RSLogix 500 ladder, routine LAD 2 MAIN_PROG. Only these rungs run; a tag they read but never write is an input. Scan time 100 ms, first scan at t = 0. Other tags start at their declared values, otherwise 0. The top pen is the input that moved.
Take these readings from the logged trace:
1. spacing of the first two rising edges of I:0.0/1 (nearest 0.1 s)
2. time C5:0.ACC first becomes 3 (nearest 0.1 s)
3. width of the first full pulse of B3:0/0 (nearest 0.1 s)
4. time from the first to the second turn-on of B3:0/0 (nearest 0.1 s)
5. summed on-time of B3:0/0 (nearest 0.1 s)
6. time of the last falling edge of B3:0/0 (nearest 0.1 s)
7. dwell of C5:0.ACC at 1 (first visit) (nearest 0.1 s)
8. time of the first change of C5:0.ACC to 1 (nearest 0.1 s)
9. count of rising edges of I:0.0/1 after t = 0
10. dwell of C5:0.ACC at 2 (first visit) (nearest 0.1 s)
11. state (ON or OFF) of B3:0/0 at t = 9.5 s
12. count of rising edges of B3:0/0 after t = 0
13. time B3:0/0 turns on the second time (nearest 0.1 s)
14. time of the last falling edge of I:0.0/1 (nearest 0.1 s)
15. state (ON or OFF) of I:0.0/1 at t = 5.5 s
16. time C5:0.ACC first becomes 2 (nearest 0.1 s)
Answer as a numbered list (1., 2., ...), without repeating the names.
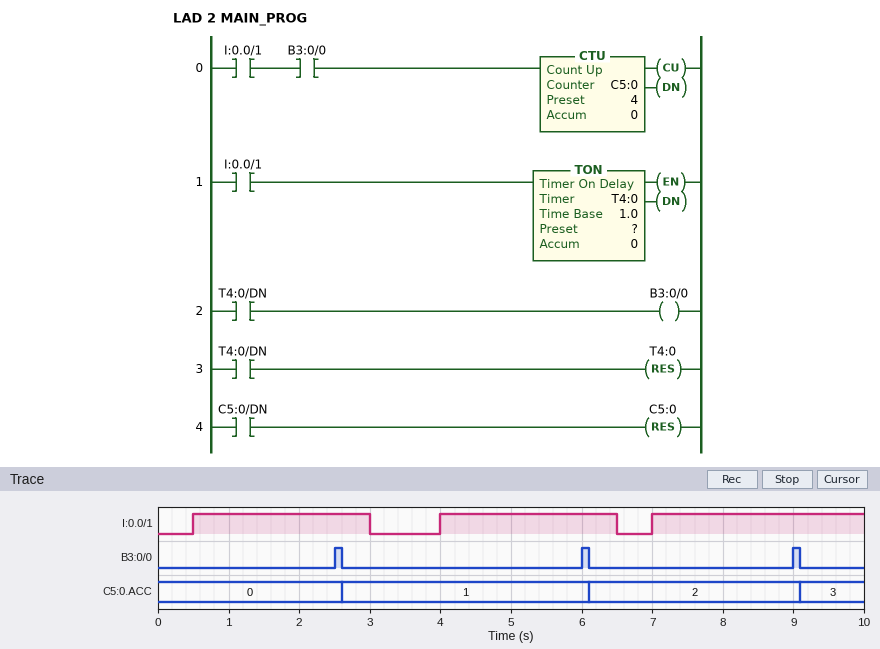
1. 3.5 s
2. 9.1 s
3. 0.1 s
4. 3.5 s
5. 0.3 s
6. 9.1 s
7. 3.5 s
8. 2.6 s
9. 3
10. 3.0 s
11. OFF
12. 3
13. 6.0 s
14. 6.5 s
15. ON
16. 6.1 s
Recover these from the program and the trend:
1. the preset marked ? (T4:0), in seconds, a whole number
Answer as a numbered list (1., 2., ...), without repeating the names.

1. 2 s
